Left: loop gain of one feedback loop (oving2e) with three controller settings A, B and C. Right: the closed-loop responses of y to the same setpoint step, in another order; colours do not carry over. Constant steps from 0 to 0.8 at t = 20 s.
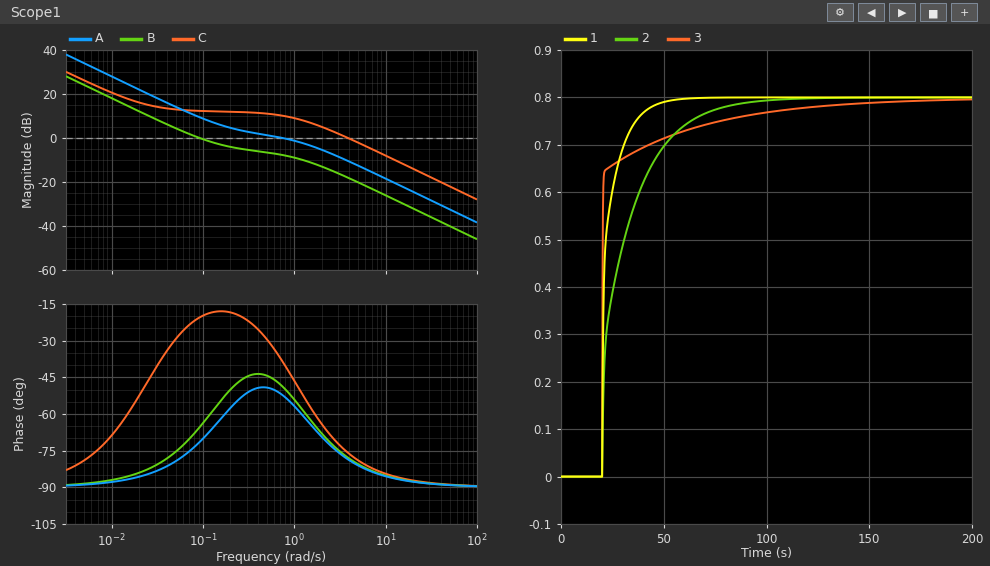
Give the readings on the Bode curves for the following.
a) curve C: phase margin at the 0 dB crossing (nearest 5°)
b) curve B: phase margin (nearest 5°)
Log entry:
105°
115°
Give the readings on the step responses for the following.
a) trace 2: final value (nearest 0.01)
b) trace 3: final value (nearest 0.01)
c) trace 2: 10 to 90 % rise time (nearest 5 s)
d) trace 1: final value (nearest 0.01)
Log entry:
0.80
0.80
35 s
0.80
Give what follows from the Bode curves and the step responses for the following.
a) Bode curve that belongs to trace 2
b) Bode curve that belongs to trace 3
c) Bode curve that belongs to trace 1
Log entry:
B
C
A
